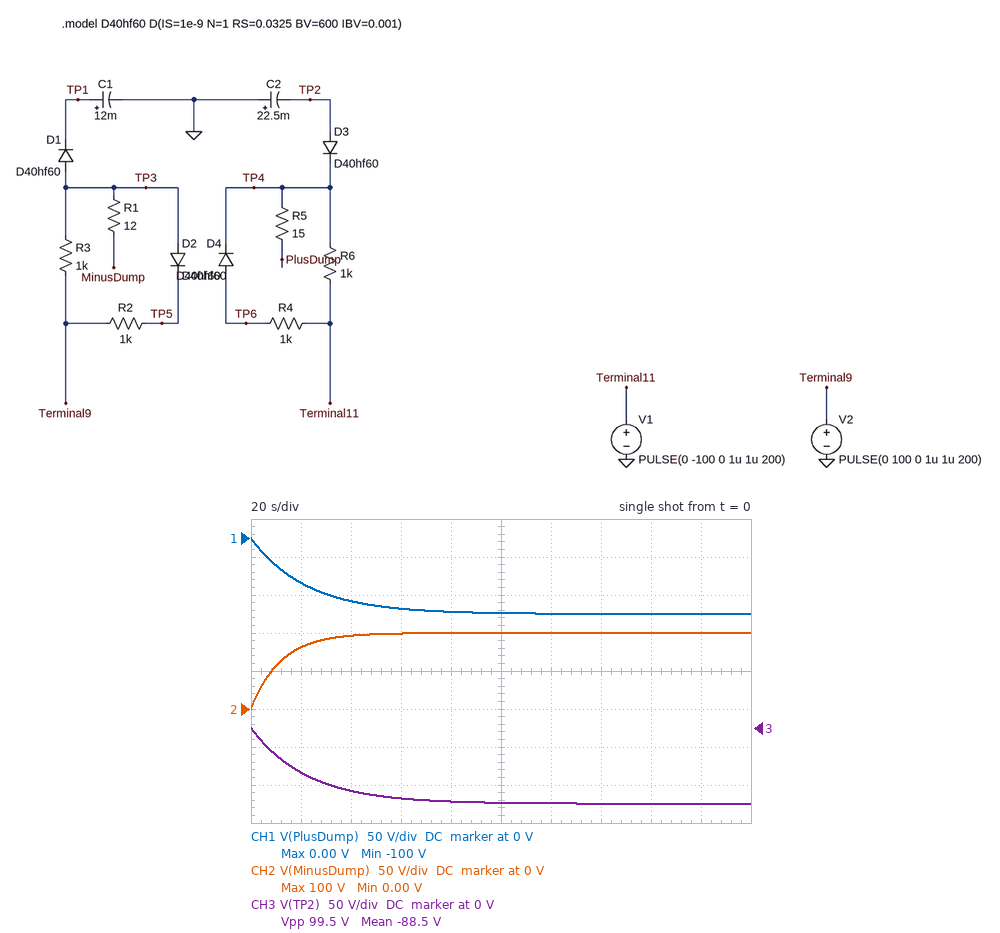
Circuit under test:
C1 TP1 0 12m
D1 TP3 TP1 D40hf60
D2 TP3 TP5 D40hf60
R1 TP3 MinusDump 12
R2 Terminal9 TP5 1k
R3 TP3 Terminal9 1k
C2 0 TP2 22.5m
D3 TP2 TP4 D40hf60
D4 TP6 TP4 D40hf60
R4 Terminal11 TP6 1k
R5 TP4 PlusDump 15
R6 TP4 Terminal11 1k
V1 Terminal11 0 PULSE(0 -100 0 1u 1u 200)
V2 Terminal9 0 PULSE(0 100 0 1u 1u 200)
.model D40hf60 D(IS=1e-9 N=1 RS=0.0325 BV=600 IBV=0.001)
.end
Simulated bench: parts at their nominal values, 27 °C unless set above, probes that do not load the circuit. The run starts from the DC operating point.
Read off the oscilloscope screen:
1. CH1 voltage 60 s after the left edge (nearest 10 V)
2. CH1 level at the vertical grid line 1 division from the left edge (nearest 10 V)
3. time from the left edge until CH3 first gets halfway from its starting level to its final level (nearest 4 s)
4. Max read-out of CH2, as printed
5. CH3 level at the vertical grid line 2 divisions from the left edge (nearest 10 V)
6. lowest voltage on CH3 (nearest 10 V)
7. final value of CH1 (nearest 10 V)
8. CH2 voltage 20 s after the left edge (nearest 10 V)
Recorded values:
-90 V
-60 V
16 s
100 V
-80 V
-100 V
-100 V
80 V
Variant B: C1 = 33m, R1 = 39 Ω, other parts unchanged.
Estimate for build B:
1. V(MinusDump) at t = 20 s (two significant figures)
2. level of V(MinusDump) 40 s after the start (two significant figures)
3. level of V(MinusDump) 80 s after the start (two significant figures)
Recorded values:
46 V
70 V
91 V
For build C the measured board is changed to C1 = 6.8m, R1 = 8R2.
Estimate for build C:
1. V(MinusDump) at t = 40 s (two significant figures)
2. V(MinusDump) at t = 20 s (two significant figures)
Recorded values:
100 V
95 V
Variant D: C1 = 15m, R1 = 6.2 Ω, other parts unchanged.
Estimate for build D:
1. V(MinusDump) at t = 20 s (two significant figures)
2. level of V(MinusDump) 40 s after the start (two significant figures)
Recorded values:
74 V
93 V
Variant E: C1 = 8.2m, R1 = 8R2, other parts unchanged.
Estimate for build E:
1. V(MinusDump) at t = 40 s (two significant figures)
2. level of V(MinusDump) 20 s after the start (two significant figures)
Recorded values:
99 V
91 V
